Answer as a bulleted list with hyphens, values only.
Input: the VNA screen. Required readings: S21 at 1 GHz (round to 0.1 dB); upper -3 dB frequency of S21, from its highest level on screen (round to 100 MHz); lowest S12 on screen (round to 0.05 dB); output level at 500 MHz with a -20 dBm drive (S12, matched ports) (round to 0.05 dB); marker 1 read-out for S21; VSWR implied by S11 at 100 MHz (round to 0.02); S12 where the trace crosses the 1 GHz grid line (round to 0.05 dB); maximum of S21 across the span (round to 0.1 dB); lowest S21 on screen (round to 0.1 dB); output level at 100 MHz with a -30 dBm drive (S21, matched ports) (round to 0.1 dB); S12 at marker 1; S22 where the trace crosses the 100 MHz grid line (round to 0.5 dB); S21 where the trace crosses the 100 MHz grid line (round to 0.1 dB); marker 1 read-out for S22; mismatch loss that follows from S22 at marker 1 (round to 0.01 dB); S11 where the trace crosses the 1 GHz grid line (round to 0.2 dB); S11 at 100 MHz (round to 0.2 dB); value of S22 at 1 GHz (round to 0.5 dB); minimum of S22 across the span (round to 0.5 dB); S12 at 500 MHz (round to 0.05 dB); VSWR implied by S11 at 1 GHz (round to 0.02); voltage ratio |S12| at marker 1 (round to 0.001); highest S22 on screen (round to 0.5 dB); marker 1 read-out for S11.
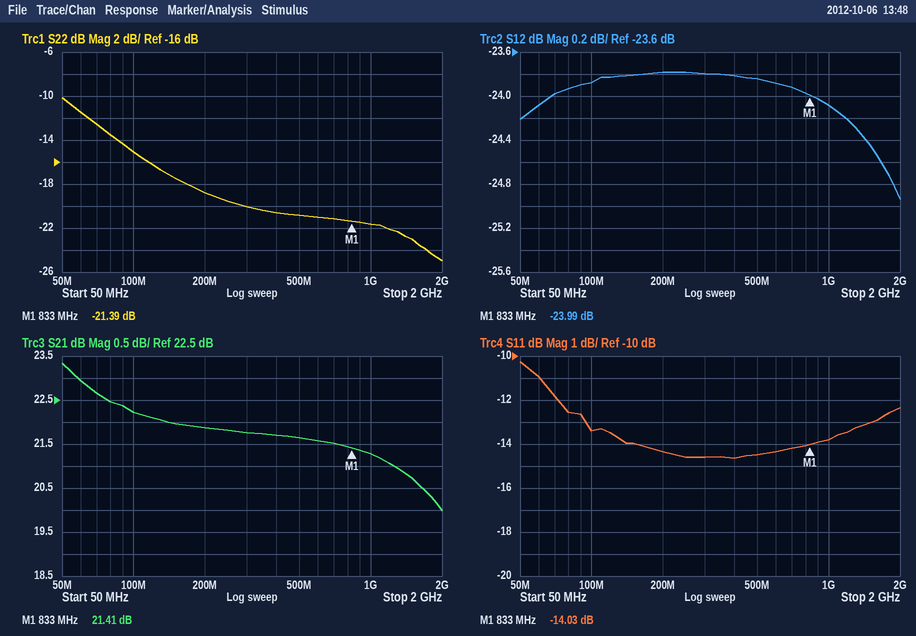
- 21.3 dB
- 1.8 GHz
- -24.95 dB
- -43.85 dBm
- 21.41 dB
- 1.54
- -24.10 dB
- 23.3 dB
- 20.0 dB
- -7.8 dBm
- -23.99 dB
- -15.0 dB
- 22.2 dB
- -21.39 dB
- 0.03 dB
- -13.8 dB
- -13.4 dB
- -21.5 dB
- -25.0 dB
- -23.85 dB
- 1.52
- 0.063
- -10.0 dB
- -14.03 dB
